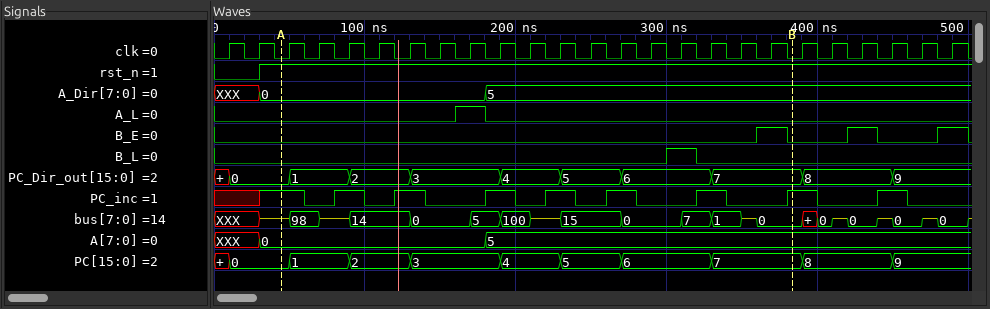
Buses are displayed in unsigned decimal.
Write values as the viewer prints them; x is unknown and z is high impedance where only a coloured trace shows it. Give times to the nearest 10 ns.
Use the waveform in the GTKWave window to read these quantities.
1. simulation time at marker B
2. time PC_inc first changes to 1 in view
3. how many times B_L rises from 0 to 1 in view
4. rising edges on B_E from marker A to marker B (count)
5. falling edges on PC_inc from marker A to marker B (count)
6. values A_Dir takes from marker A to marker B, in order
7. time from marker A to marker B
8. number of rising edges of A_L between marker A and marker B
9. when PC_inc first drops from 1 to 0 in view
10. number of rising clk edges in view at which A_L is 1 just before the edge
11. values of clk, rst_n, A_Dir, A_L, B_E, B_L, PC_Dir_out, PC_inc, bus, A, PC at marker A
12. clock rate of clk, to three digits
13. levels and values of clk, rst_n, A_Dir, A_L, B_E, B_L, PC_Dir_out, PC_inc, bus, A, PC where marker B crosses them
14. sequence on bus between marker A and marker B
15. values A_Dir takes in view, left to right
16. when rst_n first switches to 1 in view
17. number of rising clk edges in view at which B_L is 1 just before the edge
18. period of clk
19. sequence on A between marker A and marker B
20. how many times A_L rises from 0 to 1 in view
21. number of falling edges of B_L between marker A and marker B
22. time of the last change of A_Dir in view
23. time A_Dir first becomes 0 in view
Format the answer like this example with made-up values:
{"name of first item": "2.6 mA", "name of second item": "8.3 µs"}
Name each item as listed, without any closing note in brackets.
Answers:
{"simulation time at marker B": "380 ns", "time PC_inc first changes to 1 in view": "30 ns", "how many times B_L rises from 0 to 1 in view": "1", "rising edges on B_E from marker A to marker B": "1", "falling edges on PC_inc from marker A to marker B": "7", "values A_Dir takes from marker A to marker B, in order": "0, 5", "time from marker A to marker B": "340 ns", "number of rising edges of A_L between marker A and marker B": "1", "when PC_inc first drops from 1 to 0 in view": "60 ns", "number of rising clk edges in view at which A_L is 1 just before the edge": "1", "values of clk, rst_n, A_Dir, A_L, B_E, B_L, PC_Dir_out, PC_inc, bus, A, PC at marker A": "clk=0, rst_n=1, A_Dir=0, A_L=0, B_E=0, B_L=0, PC_Dir_out=0, PC_inc=1, bus=z, A=0, PC=0", "clock rate of clk, to three digits": "50.0 MHz", "levels and values of clk, rst_n, A_Dir, A_L, B_E, B_L, PC_Dir_out, PC_inc, bus, A, PC where marker B crosses them": "clk=0, rst_n=1, A_Dir=5, A_L=0, B_E=0, B_L=0, PC_Dir_out=7, PC_inc=1, bus=0, A=5, PC=7", "sequence on bus between marker A and marker B": "z, 98, z, 14, 0, 5, 100, z, 15, 0, 7, 1, z, 0", "values A_Dir takes in view, left to right": "XXX, 0, 5", "when rst_n first switches to 1 in view": "30 ns", "number of rising clk edges in view at which B_L is 1 just before the edge": "1", "period of clk": "20 ns", "sequence on A between marker A and marker B": "0, 5", "how many times A_L rises from 0 to 1 in view": "1", "number of falling edges of B_L between marker A and marker B": "1", "time of the last change of A_Dir in view": "180 ns", "time A_Dir first becomes 0 in view": "30 ns"}
